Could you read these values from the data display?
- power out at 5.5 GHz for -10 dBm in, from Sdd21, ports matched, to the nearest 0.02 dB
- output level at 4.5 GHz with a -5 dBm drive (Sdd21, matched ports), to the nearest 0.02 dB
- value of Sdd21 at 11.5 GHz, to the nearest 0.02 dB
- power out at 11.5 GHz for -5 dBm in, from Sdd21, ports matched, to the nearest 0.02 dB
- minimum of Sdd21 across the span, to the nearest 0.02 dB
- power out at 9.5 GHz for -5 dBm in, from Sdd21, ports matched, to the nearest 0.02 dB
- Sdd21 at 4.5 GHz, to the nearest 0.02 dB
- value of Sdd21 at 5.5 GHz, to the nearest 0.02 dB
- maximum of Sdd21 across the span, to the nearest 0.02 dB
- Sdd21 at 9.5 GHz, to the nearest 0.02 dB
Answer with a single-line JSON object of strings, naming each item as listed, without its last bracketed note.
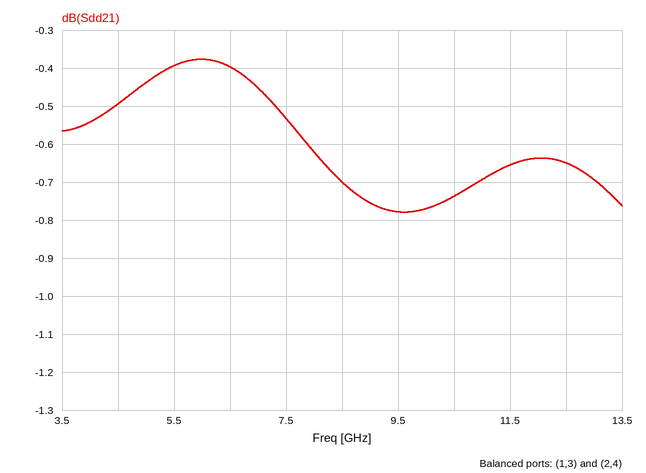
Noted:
{"power out at 5.5 GHz for -10 dBm in, from Sdd21, ports matched, to the nearest 0.02 dB": "-10.40 dBm", "output level at 4.5 GHz with a -5 dBm drive (Sdd21, matched ports), to the nearest 0.02 dB": "-5.50 dBm", "value of Sdd21 at 11.5 GHz, to the nearest 0.02 dB": "-0.66 dB", "power out at 11.5 GHz for -5 dBm in, from Sdd21, ports matched, to the nearest 0.02 dB": "-5.66 dBm", "minimum of Sdd21 across the span, to the nearest 0.02 dB": "-0.78 dB", "power out at 9.5 GHz for -5 dBm in, from Sdd21, ports matched, to the nearest 0.02 dB": "-5.78 dBm", "Sdd21 at 4.5 GHz, to the nearest 0.02 dB": "-0.50 dB", "value of Sdd21 at 5.5 GHz, to the nearest 0.02 dB": "-0.40 dB", "maximum of Sdd21 across the span, to the nearest 0.02 dB": "-0.38 dB", "Sdd21 at 9.5 GHz, to the nearest 0.02 dB": "-0.78 dB"}
